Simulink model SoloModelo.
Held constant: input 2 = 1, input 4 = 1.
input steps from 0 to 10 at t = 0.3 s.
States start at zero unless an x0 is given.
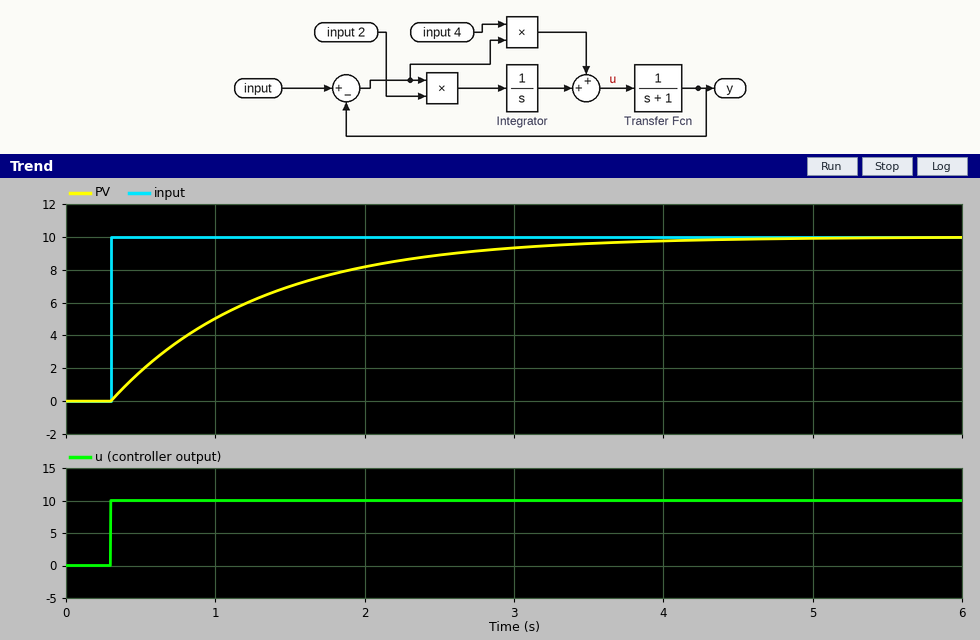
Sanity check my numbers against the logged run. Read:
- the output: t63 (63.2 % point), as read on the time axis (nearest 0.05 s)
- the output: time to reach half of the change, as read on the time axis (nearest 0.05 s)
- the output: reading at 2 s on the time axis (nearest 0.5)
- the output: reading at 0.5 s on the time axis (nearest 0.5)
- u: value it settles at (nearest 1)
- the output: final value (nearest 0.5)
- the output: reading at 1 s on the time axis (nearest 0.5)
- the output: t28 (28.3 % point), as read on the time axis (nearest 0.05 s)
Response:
1.30 s
1.00 s
8.0
2.0
10
10.0
5.0
0.65 s
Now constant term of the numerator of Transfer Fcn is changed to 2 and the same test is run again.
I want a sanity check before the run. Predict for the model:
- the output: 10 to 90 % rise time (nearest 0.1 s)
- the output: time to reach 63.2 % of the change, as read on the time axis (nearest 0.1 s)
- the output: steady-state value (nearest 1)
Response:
1.1 s
0.8 s
10
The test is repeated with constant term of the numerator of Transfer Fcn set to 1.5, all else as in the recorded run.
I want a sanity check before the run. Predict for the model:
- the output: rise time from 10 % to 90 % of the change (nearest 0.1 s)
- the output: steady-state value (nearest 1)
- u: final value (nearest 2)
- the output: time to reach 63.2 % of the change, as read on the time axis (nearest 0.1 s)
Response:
1.5 s
10
6
1.0 s
